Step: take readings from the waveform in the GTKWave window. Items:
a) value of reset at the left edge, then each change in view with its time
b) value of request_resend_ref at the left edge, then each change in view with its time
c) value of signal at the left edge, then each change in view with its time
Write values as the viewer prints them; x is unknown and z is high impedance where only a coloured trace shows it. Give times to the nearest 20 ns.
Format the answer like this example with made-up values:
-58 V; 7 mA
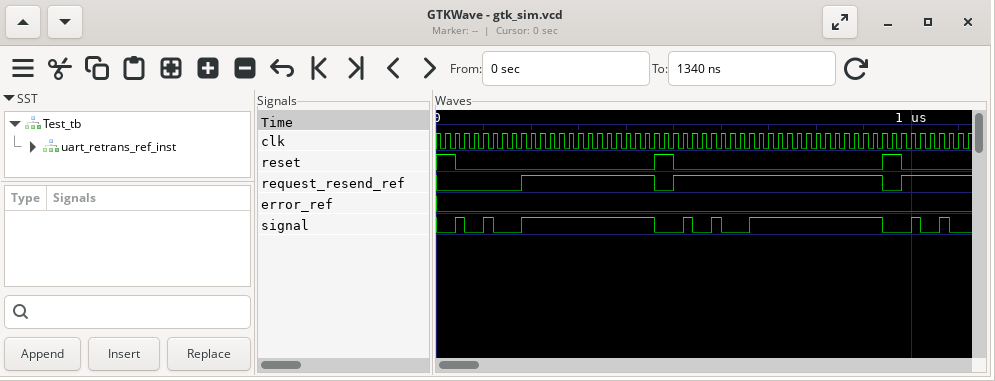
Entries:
1, 0 at 40 ns, 1 at 460 ns, 0 at 500 ns, 1 at 940 ns, 0 at 980 ns; 0, 1 at 180 ns, 0 at 460 ns, 1 at 500 ns, 0 at 940 ns, 1 at 980 ns; 0, 1 at 40 ns, 0 at 60 ns, 1 at 100 ns, 0 at 120 ns, 1 at 180 ns, 0 at 460 ns, 1 at 520 ns, 0 at 540 ns, 1 at 580 ns, 0 at 600 ns, 1 at 660 ns, 0 at 940 ns, 1 at 1000 ns, 0 at 1020 ns, 1 at 1060 ns, 0 at 1080 ns
